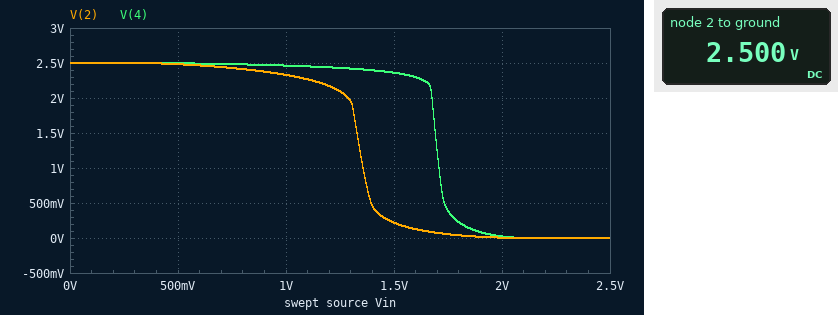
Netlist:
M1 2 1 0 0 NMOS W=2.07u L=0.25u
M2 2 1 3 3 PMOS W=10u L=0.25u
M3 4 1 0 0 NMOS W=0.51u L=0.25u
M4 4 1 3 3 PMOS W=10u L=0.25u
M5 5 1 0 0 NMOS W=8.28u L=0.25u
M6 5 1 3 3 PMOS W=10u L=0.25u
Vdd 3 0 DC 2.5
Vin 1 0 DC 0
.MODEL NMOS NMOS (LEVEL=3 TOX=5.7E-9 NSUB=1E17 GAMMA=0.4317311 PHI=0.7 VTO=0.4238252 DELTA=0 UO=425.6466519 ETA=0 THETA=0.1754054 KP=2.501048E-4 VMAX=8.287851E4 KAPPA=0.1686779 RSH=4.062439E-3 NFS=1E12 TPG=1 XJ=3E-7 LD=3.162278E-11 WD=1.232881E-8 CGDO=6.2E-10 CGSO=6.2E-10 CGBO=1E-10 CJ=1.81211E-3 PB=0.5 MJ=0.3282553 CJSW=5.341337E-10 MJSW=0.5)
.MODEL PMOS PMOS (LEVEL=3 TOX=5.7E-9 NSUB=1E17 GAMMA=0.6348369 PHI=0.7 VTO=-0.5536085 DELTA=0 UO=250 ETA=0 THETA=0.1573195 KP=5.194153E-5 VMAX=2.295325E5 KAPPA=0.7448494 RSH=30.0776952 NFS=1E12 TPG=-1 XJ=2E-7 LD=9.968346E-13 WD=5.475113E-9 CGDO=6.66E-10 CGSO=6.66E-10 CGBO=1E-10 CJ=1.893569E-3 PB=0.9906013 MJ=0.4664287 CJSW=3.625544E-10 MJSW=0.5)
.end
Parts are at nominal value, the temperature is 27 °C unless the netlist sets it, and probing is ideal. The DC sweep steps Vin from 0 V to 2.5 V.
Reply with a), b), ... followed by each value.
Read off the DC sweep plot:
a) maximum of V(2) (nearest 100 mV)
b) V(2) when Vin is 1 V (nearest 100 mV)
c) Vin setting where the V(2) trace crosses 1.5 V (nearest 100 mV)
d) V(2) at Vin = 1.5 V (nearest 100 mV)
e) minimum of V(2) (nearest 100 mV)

a) 2.5 V
b) 2.3 V
c) 1.3 V
d) 200 mV
e) 0 V
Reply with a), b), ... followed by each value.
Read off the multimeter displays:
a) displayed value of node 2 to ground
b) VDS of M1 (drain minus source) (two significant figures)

a) 2.500 V
b) 2.5 V
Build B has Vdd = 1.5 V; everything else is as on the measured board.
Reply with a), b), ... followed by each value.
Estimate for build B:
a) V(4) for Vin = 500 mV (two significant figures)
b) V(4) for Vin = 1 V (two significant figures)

a) 1.5 V
b) 50 mV
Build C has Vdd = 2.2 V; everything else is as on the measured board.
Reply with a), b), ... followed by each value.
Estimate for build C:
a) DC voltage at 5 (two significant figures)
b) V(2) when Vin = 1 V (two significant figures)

a) 2.2 V
b) 2.0 V
